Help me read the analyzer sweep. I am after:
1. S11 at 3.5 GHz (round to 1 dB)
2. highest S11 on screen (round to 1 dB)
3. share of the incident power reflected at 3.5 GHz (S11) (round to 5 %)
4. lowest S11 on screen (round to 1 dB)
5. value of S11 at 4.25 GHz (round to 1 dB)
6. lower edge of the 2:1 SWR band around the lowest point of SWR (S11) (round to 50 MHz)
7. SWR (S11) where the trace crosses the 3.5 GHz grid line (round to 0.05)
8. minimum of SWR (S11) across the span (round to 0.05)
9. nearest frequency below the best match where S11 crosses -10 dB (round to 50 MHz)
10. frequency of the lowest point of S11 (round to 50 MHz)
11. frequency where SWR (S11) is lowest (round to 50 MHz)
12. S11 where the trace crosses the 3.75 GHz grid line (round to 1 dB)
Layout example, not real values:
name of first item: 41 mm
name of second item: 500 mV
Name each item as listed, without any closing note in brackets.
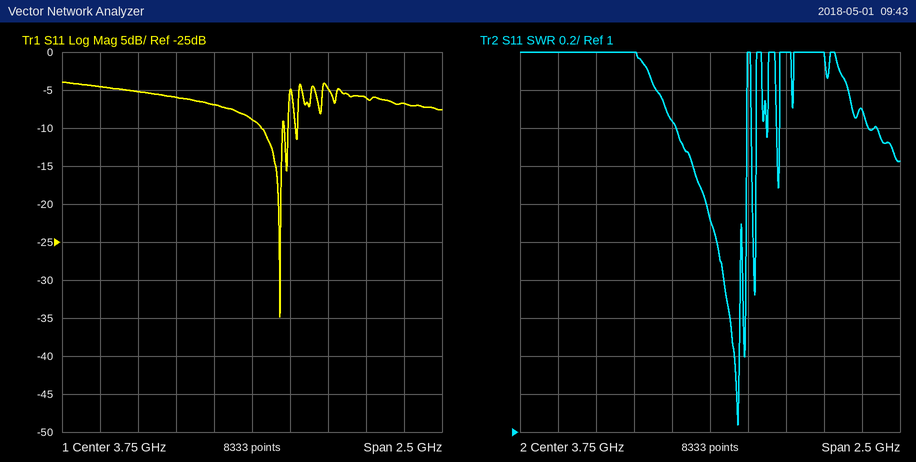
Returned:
S11 at 3.5 GHz: -7 dB
highest S11 on screen: -4 dB
share of the incident power reflected at 3.5 GHz (S11): 20 %
lowest S11 on screen: -35 dB
value of S11 at 4.25 GHz: -5 dB
lower edge of the 2:1 SWR band around the lowest point of SWR (S11): 3.80 GHz
SWR (S11) where the trace crosses the 3.5 GHz grid line: 2.65
minimum of SWR (S11) across the span: 1.05
nearest frequency below the best match where S11 crosses -10 dB: 3.80 GHz
frequency of the lowest point of S11: 3.95 GHz
frequency where SWR (S11) is lowest: 3.95 GHz
S11 where the trace crosses the 3.75 GHz grid line: -9 dB
